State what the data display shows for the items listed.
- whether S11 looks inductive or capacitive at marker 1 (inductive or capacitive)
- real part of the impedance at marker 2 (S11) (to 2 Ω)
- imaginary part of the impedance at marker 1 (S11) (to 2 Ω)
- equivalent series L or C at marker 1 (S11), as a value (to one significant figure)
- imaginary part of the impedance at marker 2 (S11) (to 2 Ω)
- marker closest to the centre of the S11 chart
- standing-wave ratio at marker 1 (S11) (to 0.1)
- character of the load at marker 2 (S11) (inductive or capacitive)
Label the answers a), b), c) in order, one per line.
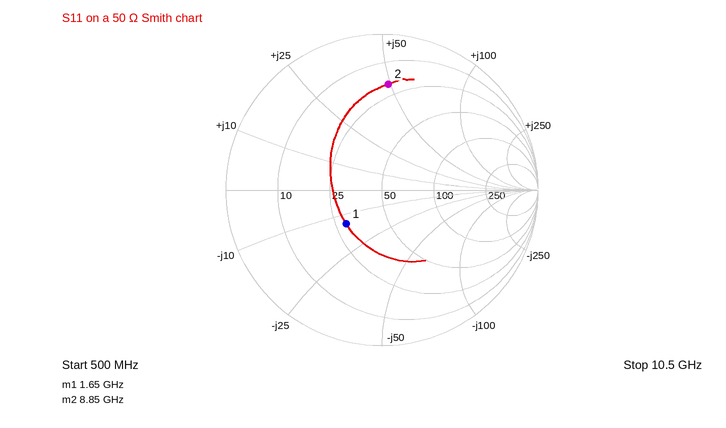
a) capacitive
b) 20 Ω
c) -14 Ω
d) 7 pF
e) +50 Ω
f) marker 1
g) 1.9
h) inductive
